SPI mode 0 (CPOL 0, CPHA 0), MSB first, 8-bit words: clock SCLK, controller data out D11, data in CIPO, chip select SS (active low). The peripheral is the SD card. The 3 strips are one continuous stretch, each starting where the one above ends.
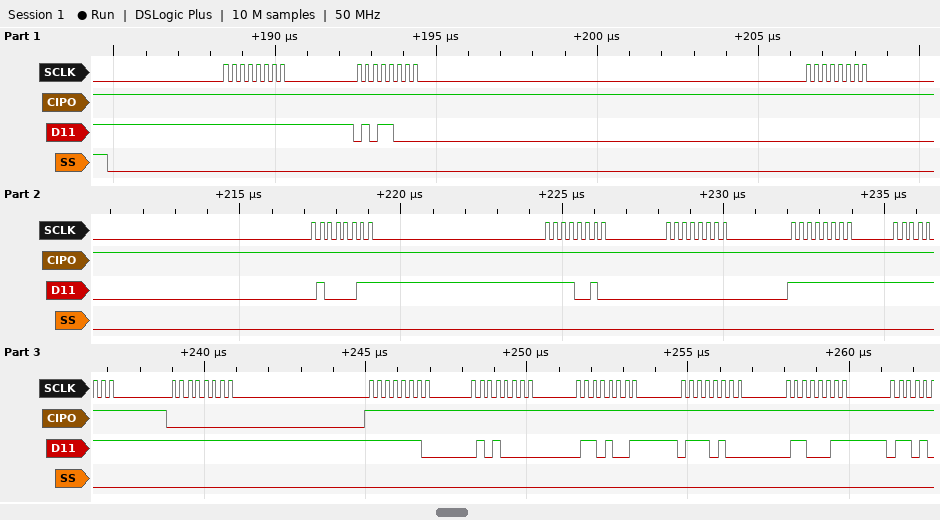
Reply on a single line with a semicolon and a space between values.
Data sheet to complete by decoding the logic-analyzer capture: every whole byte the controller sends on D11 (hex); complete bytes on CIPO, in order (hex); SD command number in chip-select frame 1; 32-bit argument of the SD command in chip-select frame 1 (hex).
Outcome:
FF 58 00 43 F2 00 FF FF FF FE 50 69 74 63; FF FF FF FF FF FF FF FF 00 FF FF FF FF FF; CMD24; 0x0043F200
